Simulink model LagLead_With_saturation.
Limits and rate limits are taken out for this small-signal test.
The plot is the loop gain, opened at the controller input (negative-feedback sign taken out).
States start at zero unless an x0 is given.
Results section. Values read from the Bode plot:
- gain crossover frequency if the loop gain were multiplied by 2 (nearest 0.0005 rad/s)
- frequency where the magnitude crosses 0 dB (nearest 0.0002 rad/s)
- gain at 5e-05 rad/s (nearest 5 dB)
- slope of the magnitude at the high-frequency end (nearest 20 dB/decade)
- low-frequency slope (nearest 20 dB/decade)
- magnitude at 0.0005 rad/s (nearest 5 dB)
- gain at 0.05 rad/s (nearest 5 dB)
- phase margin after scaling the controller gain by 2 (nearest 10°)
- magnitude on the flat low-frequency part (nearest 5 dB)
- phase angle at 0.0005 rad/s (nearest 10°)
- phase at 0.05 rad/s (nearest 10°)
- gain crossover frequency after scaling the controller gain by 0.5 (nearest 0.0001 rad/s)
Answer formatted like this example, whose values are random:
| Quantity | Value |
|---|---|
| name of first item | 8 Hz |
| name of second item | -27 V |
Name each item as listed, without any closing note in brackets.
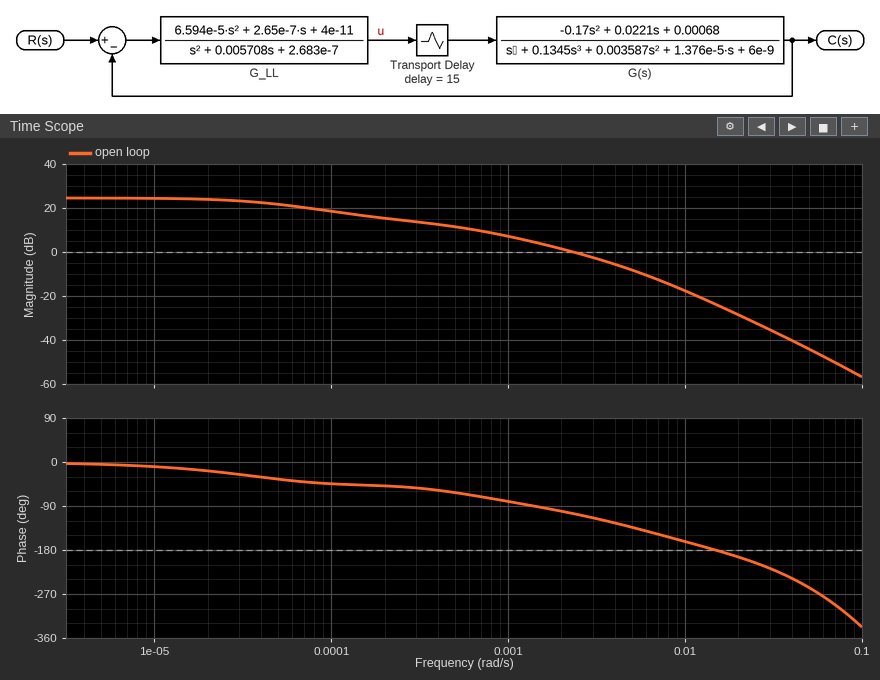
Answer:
| Quantity | Value |
|---|---|
| gain crossover frequency if the loop gain were multiplied by 2 | 0.0040 rad/s |
| frequency where the magnitude crosses 0 dB | 0.0024 rad/s |
| gain at 5e-05 rad/s | 20 dB |
| slope of the magnitude at the high-frequency end | -40 dB/decade |
| low-frequency slope | 0 dB/decade |
| magnitude at 0.0005 rad/s | 10 dB |
| gain at 0.05 rad/s | -45 dB |
| phase margin after scaling the controller gain by 2 | 50° |
| magnitude on the flat low-frequency part | 25 dB |
| phase angle at 0.0005 rad/s | -60° |
| phase at 0.05 rad/s | -260° |
| gain crossover frequency after scaling the controller gain by 0.5 | 0.0012 rad/s |
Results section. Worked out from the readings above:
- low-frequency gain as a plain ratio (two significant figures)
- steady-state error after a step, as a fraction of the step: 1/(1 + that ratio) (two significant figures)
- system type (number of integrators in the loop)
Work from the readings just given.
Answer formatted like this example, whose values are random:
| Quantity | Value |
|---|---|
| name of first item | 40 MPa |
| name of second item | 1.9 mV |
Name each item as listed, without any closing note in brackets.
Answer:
| Quantity | Value |
|---|---|
| low-frequency gain as a plain ratio | 18 |
| steady-state error after a step, as a fraction of the step: 1/(1 + that ratio) | 0.053 |
| system type | 0 |
